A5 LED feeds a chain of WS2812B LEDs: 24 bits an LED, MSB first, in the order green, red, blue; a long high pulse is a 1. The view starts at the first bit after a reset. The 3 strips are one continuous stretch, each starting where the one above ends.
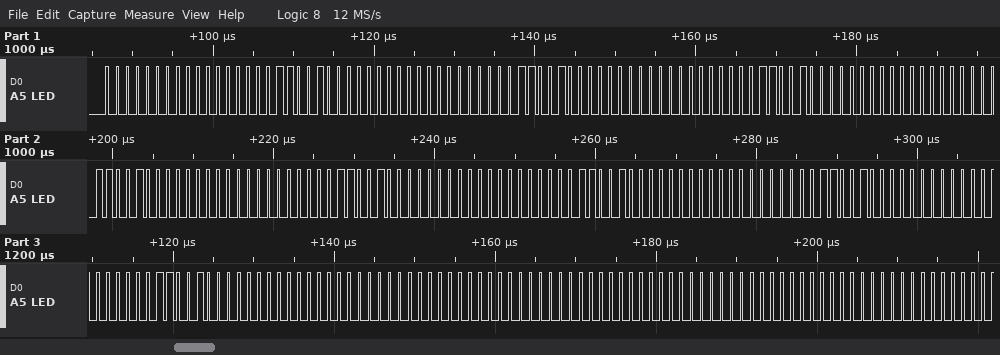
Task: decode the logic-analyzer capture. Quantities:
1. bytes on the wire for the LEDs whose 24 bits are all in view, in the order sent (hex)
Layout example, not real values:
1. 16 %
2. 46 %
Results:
1. 00 00 64 00 00 64 00 00 64 00 00 64 00 00 64 00 00 64 00 00 64 00 00 64 00 00 00 00 00 00 00 00 00
